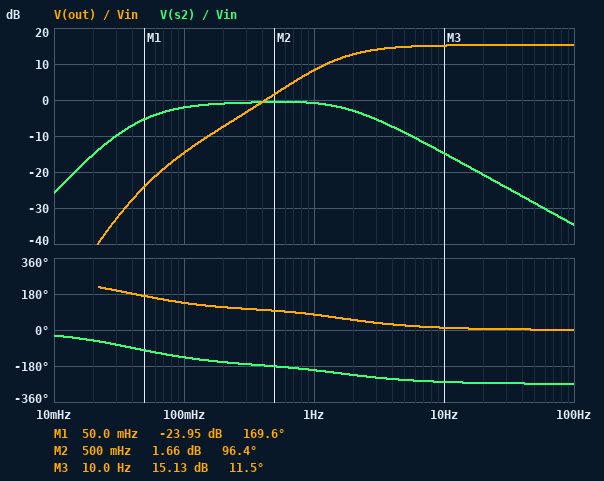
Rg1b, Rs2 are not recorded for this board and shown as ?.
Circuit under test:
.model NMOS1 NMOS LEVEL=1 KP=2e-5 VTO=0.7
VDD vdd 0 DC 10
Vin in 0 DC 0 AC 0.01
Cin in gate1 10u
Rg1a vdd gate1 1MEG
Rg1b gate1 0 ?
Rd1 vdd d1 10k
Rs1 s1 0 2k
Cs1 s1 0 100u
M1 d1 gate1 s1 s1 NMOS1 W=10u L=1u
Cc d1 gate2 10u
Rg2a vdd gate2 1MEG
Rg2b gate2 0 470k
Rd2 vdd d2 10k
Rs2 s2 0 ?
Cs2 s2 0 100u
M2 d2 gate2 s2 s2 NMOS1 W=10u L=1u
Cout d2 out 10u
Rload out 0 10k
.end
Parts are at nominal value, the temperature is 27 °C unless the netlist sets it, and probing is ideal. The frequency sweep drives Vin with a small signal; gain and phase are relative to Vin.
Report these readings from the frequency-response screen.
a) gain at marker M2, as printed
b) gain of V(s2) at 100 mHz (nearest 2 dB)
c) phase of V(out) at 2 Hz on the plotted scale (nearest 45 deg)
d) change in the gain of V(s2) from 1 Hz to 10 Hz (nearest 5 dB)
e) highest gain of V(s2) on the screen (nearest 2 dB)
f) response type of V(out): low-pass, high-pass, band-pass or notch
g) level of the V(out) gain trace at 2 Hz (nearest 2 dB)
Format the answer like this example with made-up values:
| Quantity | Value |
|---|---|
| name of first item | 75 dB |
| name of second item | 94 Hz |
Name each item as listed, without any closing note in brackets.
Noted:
| Quantity | Value |
|---|---|
| gain at marker M2, as printed | 1.66 dB |
| gain of V(s2) at 100 mHz | -2 dB |
| phase of V(out) at 2 Hz on the plotted scale | 45 deg |
| change in the gain of V(s2) from 1 Hz to 10 Hz | -15 dB |
| highest gain of V(s2) on the screen | 0 dB |
| response type of V(out): low-pass, high-pass, band-pass or notch | high-pass |
| level of the V(out) gain trace at 2 Hz | 12 dB |
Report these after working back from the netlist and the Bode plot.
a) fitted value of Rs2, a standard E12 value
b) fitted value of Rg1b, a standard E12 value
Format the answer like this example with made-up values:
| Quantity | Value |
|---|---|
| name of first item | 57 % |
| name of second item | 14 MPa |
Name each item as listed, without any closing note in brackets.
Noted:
| Quantity | Value |
|---|---|
| fitted value of Rs2, a standard E12 value | 2.7 kΩ |
| fitted value of Rg1b, a standard E12 value | 820 kΩ |
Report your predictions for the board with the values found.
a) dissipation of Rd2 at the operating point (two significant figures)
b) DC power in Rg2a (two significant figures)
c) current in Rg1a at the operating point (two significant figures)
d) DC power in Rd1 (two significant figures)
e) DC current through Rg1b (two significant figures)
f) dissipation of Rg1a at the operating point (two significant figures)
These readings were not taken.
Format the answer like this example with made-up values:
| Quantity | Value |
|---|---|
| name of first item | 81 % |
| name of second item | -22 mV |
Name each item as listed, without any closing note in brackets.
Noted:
| Quantity | Value |
|---|---|
| dissipation of Rd2 at the operating point | 850 µW |
| DC power in Rg2a | 46 µW |
| current in Rg1a at the operating point | 5.5 µA |
| DC power in Rd1 | 4.1 mW |
| DC current through Rg1b | 5.5 µA |
| dissipation of Rg1a at the operating point | 30 µW |
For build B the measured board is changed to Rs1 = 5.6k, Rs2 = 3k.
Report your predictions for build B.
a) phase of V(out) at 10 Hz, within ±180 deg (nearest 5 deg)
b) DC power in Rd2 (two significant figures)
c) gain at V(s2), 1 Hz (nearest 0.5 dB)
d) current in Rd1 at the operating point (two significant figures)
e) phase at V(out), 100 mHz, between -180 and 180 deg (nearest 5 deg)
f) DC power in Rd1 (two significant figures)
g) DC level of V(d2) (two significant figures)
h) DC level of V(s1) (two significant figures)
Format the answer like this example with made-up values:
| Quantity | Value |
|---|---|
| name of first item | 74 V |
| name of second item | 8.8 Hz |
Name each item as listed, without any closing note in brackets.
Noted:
| Quantity | Value |
|---|---|
| phase of V(out) at 10 Hz, within ±180 deg | 10 deg |
| DC power in Rd2 | 770 µW |
| gain at V(s2), 1 Hz | 0 dB |
| current in Rd1 at the operating point | 350 µA |
| phase at V(out), 100 mHz, between -180 and 180 deg | 145 deg |
| DC power in Rd1 | 1.2 mW |
| DC level of V(d2) | 7.2 V |
| DC level of V(s1) | 1.9 V |
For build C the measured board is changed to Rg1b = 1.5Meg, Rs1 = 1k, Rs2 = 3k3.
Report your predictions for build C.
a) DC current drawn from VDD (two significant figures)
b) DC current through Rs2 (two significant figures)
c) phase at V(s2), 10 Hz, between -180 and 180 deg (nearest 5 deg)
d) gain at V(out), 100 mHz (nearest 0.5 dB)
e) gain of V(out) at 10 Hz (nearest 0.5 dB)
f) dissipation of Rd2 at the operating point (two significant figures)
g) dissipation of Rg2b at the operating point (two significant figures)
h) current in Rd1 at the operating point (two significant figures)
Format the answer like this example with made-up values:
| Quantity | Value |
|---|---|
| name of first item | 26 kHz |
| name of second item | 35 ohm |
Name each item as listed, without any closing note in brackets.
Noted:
| Quantity | Value |
|---|---|
| DC current drawn from VDD | 1.1 mA |
| DC current through Rs2 | 260 µA |
| phase at V(s2), 10 Hz, between -180 and 180 deg | 95 deg |
| gain at V(out), 100 mHz | -34.0 dB |
| gain of V(out) at 10 Hz | -7.5 dB |
| dissipation of Rd2 at the operating point | 700 µW |
| dissipation of Rg2b at the operating point | 22 µW |
| current in Rd1 at the operating point | 820 µA |
